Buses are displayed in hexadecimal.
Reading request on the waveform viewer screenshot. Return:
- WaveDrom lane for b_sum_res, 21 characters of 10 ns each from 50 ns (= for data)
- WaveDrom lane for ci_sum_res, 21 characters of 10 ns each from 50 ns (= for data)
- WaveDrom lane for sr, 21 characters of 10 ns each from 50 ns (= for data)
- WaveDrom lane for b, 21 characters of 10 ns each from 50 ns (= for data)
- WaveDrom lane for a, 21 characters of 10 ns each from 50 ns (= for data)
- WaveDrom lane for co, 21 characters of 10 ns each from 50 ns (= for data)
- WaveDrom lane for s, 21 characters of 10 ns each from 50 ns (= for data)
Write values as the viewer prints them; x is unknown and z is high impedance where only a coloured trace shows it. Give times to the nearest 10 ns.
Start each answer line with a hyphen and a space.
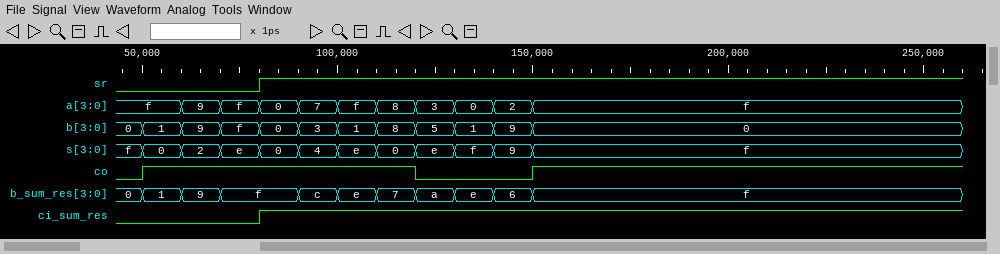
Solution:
- {name: 'b_sum_res', wave: '===.=======..........', data: '1 9 f c e 7 a e 6 f'}
- {name: 'ci_sum_res', wave: '0..1.................'}
- {name: 'sr', wave: '0..1.................'}
- {name: 'b', wave: '===========..........', data: '1 9 f 0 3 1 8 5 1 9 0'}
- {name: 'a', wave: '===========..........', data: 'f 9 f 0 7 f 8 3 0 2 f'}
- {name: 'co', wave: '1......0..1..........'}
- {name: 's', wave: '===========..........', data: '0 2 e 0 4 e 0 e f 9 f'}
